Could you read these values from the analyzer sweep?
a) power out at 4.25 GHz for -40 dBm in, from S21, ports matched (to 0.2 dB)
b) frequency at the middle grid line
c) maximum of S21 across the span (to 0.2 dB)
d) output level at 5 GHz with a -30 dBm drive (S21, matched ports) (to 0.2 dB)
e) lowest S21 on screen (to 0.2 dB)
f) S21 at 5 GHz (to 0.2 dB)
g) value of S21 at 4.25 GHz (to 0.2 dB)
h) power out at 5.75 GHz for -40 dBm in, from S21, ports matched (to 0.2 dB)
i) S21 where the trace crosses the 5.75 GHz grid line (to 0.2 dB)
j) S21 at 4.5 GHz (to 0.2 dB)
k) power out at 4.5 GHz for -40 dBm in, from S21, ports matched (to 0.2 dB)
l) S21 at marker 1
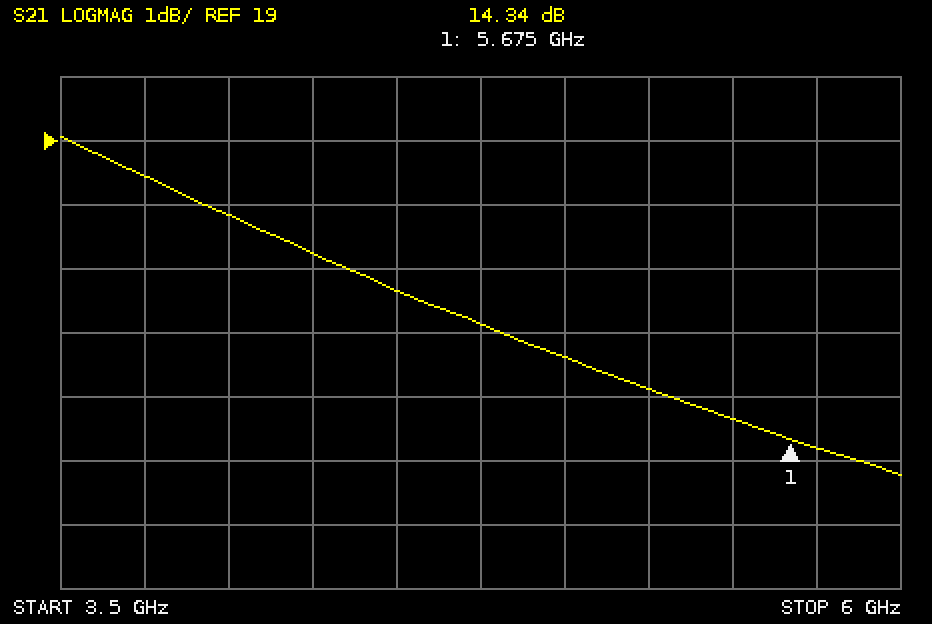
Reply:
-22.8 dBm
4.75 GHz
19.0 dB
-14.4 dBm
13.8 dB
15.6 dB
17.2 dB
-25.8 dBm
14.2 dB
16.6 dB
-23.4 dBm
14.34 dB
